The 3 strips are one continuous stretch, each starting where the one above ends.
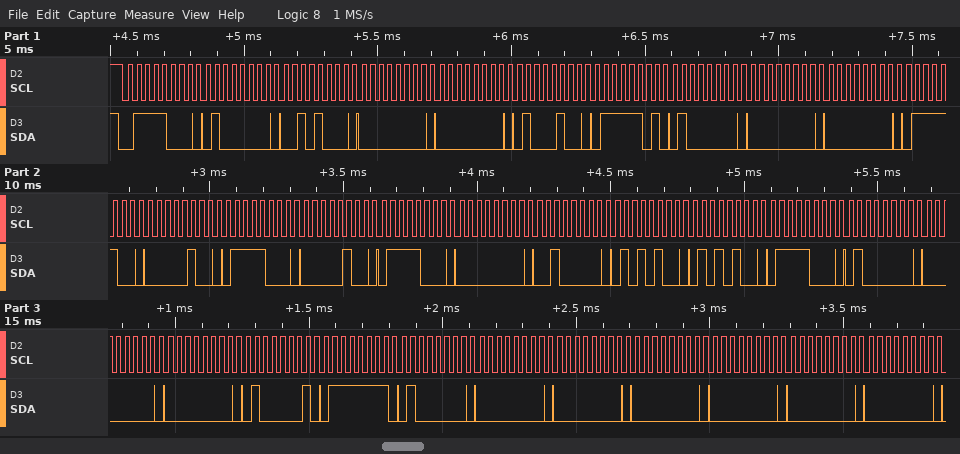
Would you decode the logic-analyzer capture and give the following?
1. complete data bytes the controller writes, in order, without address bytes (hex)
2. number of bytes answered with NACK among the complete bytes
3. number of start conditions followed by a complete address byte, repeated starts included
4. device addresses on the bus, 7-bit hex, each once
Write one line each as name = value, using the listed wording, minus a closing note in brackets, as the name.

complete data bytes the controller writes, in order, without address bytes = 40 28 00 00 44 7D 40 00 00 7C 04 78 04 78 00 20 54 54 78 40 00 00 41 7F 40 00 00 00 00 00 00
number of bytes answered with NACK among the complete bytes = 0
number of start conditions followed by a complete address byte, repeated starts included = 1
device addresses on the bus, 7-bit hex, each once = 0x3C
